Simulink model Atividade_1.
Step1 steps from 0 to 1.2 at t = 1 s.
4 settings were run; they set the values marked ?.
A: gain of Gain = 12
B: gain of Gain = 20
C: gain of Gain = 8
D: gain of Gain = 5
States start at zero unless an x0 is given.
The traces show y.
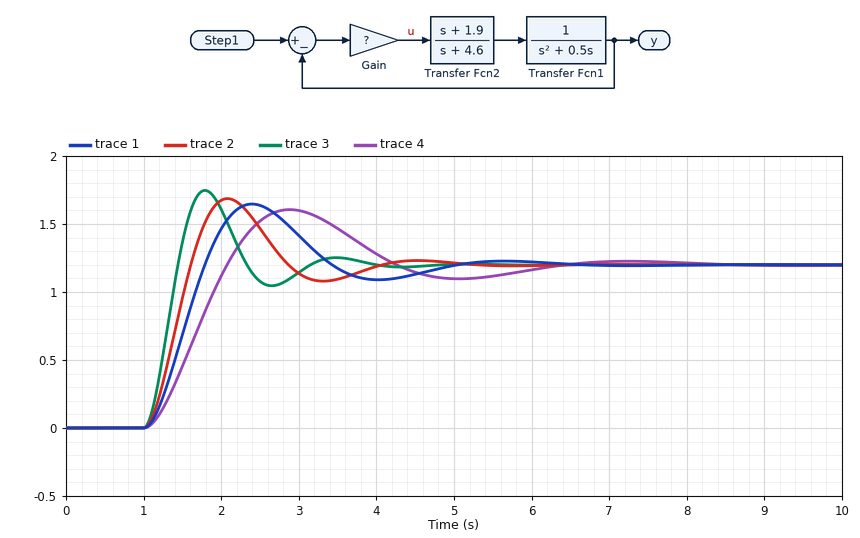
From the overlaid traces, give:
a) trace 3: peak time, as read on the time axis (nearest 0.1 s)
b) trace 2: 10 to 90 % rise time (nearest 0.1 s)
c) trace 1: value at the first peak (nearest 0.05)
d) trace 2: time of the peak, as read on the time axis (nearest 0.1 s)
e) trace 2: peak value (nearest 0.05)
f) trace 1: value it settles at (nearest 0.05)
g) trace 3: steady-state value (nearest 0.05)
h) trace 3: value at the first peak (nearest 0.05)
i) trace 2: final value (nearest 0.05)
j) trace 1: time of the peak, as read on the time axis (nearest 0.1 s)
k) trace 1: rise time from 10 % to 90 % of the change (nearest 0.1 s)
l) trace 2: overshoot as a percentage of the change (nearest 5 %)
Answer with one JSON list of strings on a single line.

["1.8 s", "0.4 s", "1.65", "2.1 s", "1.70", "1.20", "1.20", "1.75", "1.20", "2.4 s", "0.5 s", "40 %"]
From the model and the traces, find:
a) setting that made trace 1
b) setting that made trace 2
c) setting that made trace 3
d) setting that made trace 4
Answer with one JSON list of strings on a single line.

["C", "A", "B", "D"]
